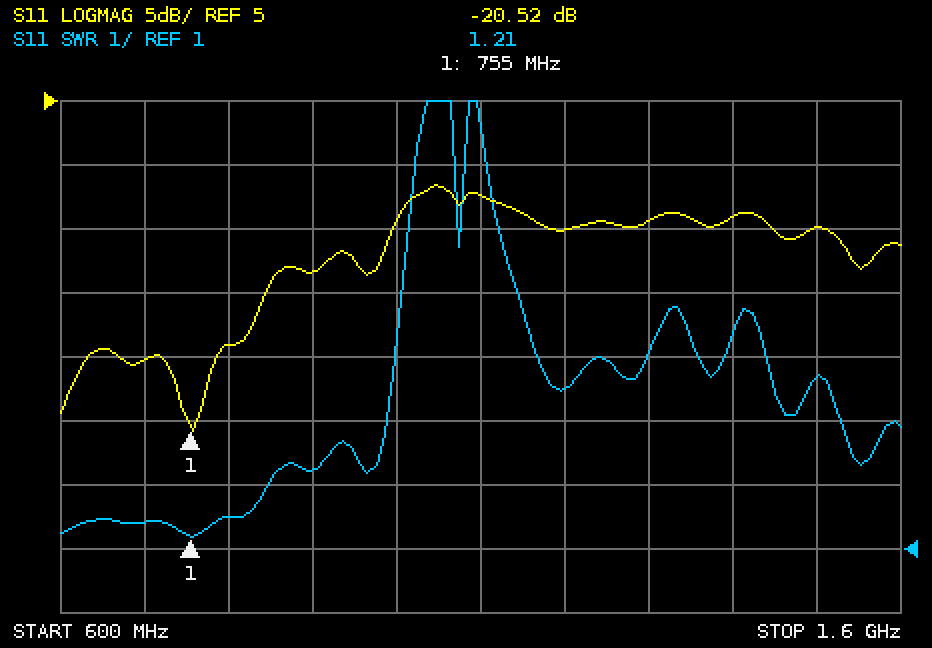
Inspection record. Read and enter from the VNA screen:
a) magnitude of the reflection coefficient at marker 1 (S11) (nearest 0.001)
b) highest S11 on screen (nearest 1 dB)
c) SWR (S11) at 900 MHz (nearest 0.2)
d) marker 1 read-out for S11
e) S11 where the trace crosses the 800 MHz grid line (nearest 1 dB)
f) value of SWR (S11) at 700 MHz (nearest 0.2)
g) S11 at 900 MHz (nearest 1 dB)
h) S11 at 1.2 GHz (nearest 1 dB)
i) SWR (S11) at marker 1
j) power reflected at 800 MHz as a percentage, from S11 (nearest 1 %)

0.094
-2 dB
2.2
-20.52 dB
-14 dB
1.4
-8 dB
-5 dB
1.21
4 %
